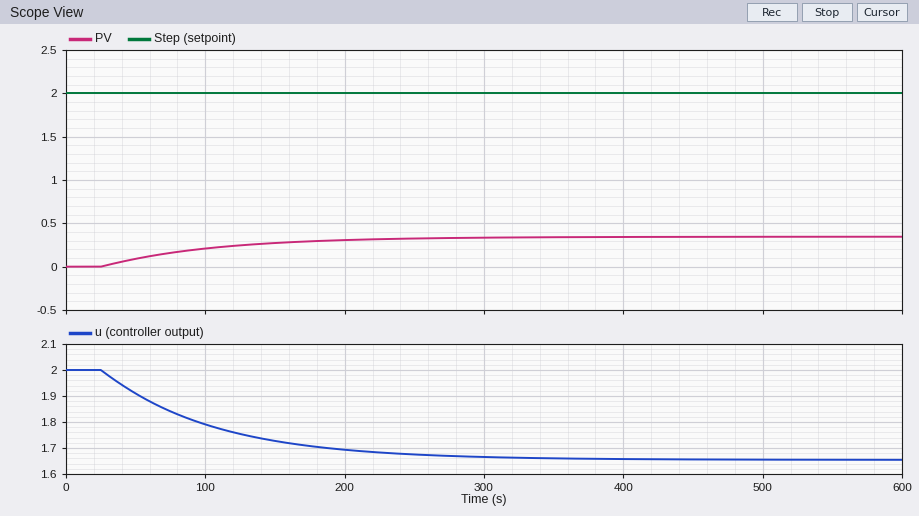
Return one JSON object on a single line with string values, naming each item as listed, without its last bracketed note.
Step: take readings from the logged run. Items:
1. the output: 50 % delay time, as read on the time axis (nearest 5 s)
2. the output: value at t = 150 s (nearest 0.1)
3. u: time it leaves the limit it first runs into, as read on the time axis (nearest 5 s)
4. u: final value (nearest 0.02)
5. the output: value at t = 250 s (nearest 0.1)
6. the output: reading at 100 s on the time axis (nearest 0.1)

{"the output: 50 % delay time, as read on the time axis": "80 s", "the output: value at t = 150 s": "0.3", "u: time it leaves the limit it first runs into, as read on the time axis": "25 s", "u: final value": "1.66", "the output: value at t = 250 s": "0.3", "the output: reading at 100 s on the time axis": "0.2"}
